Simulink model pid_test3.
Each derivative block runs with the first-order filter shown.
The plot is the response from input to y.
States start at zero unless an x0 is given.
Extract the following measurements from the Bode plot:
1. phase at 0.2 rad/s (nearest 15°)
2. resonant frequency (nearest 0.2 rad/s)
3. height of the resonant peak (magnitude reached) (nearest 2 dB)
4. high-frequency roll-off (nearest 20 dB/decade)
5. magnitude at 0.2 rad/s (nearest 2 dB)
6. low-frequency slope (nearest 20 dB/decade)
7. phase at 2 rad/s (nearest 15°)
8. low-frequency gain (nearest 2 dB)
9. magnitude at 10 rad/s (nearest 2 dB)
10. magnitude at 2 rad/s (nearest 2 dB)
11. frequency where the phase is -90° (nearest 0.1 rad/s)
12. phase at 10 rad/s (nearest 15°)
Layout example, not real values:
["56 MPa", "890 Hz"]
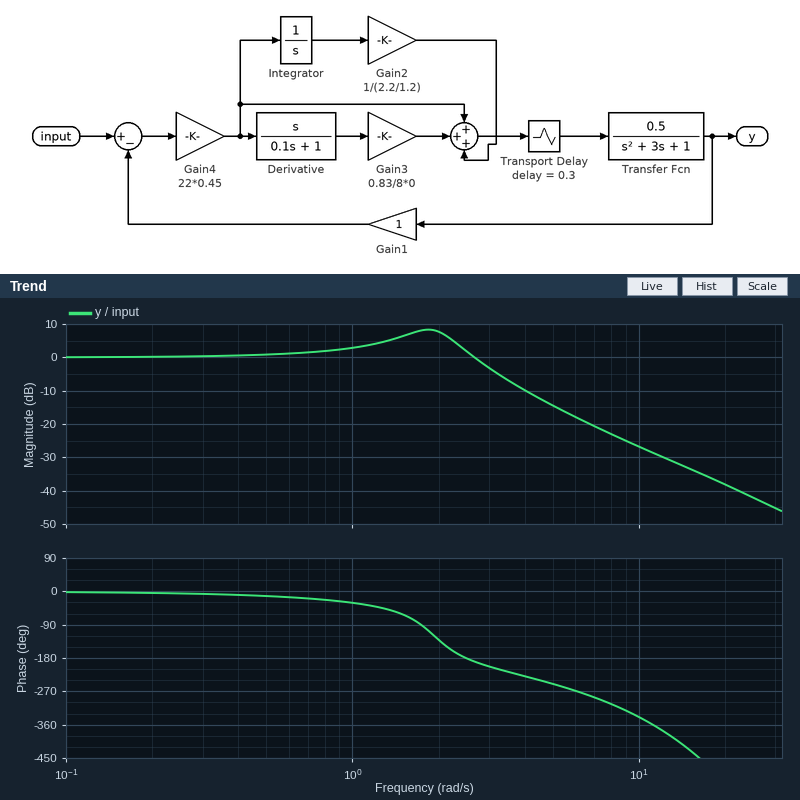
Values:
["0°", "1.8 rad/s", "8 dB", "-40 dB/decade", "0 dB", "0 dB/decade", "-135°", "0 dB", "-26 dB", "8 dB", "1.7 rad/s", "-345°"]
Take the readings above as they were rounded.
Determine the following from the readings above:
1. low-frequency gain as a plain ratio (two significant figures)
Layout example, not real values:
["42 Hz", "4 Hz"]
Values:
["1.0"]
